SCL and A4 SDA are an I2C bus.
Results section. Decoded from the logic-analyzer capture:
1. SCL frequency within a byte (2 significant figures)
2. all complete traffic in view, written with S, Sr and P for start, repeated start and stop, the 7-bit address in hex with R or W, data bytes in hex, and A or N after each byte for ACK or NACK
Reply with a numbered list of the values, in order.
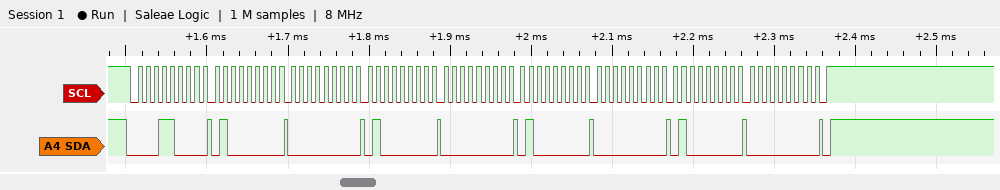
1. 100 kHz
2. S 0CW A 40 A 00 A 40 A 00 A 40 A 00 A 40 A 00 A P
